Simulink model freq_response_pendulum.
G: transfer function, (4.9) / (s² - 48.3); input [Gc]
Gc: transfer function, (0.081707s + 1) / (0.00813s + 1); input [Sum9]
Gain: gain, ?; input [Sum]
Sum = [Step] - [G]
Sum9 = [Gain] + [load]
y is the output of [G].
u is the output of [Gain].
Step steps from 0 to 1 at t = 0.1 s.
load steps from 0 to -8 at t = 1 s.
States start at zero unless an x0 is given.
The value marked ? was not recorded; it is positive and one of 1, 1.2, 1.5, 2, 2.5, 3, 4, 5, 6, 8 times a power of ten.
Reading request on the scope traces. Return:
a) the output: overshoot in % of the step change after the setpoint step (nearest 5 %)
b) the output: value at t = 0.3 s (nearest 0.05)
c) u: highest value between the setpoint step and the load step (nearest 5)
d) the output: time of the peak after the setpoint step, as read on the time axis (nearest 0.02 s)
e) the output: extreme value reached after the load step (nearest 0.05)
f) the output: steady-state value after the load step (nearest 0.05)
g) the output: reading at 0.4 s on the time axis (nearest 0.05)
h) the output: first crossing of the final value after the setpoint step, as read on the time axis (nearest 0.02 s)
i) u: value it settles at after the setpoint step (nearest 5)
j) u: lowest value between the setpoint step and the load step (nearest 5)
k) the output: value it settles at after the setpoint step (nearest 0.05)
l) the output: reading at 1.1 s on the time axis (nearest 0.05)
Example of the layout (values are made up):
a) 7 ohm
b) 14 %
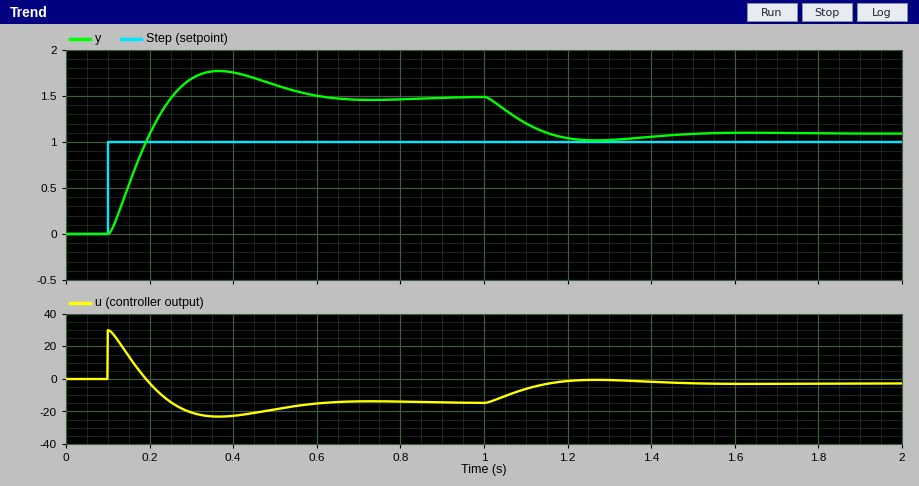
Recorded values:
a) 20 %
b) 1.70
c) 30
d) 0.36 s
e) 1.00
f) 1.10
g) 1.75
h) 0.26 s
i) -15
j) -25
k) 1.50
l) 1.20
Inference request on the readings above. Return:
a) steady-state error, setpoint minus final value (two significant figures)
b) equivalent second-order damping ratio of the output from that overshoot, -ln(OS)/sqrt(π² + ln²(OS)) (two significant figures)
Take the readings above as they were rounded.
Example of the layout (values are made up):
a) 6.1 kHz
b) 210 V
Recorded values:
a) -0.50
b) 0.46
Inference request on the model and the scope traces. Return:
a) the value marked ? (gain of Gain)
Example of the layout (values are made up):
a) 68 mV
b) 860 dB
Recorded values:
a) 30
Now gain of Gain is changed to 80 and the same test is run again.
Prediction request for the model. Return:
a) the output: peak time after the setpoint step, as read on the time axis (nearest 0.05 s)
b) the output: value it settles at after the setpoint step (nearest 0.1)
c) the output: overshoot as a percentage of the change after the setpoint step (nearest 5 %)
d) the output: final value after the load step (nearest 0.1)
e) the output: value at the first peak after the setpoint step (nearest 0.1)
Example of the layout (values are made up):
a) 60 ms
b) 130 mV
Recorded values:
a) 0.20 s
b) 1.1
c) 15 %
d) 1.0
e) 1.3
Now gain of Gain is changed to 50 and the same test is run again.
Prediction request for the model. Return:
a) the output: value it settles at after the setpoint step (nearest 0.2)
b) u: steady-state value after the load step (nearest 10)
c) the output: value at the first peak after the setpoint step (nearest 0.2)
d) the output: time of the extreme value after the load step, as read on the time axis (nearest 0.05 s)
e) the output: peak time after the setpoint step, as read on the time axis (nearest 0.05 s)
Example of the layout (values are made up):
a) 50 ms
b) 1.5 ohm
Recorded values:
a) 1.2
b) 0
c) 1.4
d) 1.15 s
e) 0.25 s
